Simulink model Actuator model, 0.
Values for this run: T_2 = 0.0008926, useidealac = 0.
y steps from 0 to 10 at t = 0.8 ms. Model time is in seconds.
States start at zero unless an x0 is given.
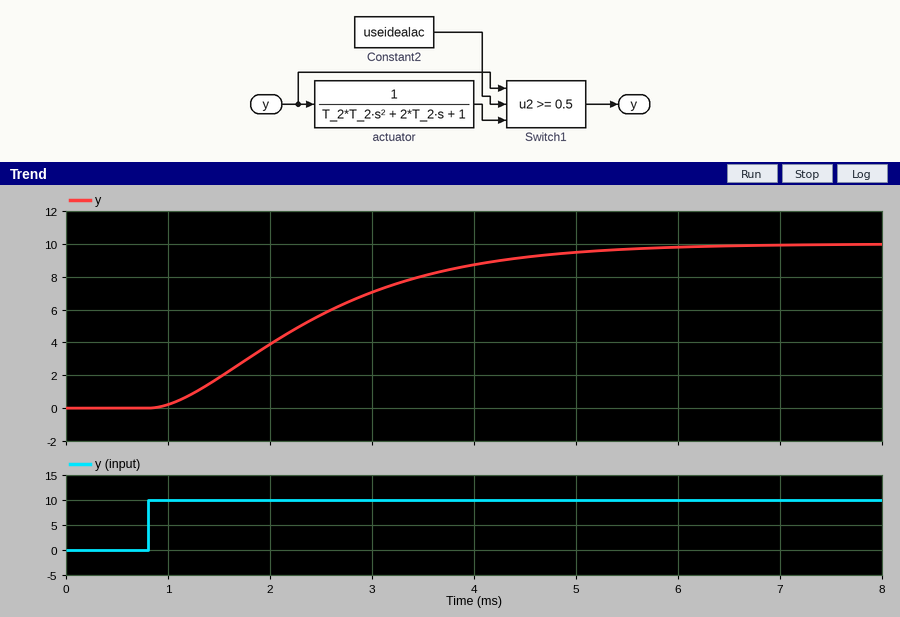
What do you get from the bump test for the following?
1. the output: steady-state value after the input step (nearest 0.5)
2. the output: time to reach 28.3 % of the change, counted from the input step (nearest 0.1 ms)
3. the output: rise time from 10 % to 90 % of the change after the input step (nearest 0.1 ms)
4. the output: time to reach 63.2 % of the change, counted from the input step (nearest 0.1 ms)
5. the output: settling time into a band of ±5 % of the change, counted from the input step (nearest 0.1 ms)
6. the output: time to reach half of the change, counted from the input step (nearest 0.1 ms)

10.0
0.9 ms
3.0 ms
1.9 ms
4.2 ms
1.5 ms
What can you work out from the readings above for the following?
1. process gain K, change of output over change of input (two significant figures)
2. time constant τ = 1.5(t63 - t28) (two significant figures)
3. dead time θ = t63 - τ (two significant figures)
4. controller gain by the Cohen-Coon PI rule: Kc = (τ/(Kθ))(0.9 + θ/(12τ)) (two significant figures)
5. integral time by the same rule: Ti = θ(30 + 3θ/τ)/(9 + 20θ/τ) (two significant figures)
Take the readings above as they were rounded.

1.0
1.5 ms
0.40 ms
3.5
0.86 ms
